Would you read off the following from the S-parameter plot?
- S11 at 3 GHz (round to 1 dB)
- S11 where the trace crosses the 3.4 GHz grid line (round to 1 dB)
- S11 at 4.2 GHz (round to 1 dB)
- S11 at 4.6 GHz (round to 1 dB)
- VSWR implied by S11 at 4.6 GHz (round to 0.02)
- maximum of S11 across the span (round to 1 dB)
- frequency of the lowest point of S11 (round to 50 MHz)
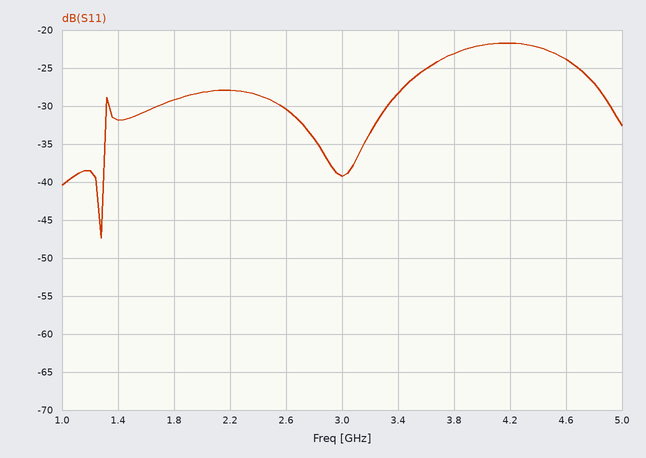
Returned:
-39 dB
-28 dB
-22 dB
-24 dB
1.14
-22 dB
1.30 GHz
